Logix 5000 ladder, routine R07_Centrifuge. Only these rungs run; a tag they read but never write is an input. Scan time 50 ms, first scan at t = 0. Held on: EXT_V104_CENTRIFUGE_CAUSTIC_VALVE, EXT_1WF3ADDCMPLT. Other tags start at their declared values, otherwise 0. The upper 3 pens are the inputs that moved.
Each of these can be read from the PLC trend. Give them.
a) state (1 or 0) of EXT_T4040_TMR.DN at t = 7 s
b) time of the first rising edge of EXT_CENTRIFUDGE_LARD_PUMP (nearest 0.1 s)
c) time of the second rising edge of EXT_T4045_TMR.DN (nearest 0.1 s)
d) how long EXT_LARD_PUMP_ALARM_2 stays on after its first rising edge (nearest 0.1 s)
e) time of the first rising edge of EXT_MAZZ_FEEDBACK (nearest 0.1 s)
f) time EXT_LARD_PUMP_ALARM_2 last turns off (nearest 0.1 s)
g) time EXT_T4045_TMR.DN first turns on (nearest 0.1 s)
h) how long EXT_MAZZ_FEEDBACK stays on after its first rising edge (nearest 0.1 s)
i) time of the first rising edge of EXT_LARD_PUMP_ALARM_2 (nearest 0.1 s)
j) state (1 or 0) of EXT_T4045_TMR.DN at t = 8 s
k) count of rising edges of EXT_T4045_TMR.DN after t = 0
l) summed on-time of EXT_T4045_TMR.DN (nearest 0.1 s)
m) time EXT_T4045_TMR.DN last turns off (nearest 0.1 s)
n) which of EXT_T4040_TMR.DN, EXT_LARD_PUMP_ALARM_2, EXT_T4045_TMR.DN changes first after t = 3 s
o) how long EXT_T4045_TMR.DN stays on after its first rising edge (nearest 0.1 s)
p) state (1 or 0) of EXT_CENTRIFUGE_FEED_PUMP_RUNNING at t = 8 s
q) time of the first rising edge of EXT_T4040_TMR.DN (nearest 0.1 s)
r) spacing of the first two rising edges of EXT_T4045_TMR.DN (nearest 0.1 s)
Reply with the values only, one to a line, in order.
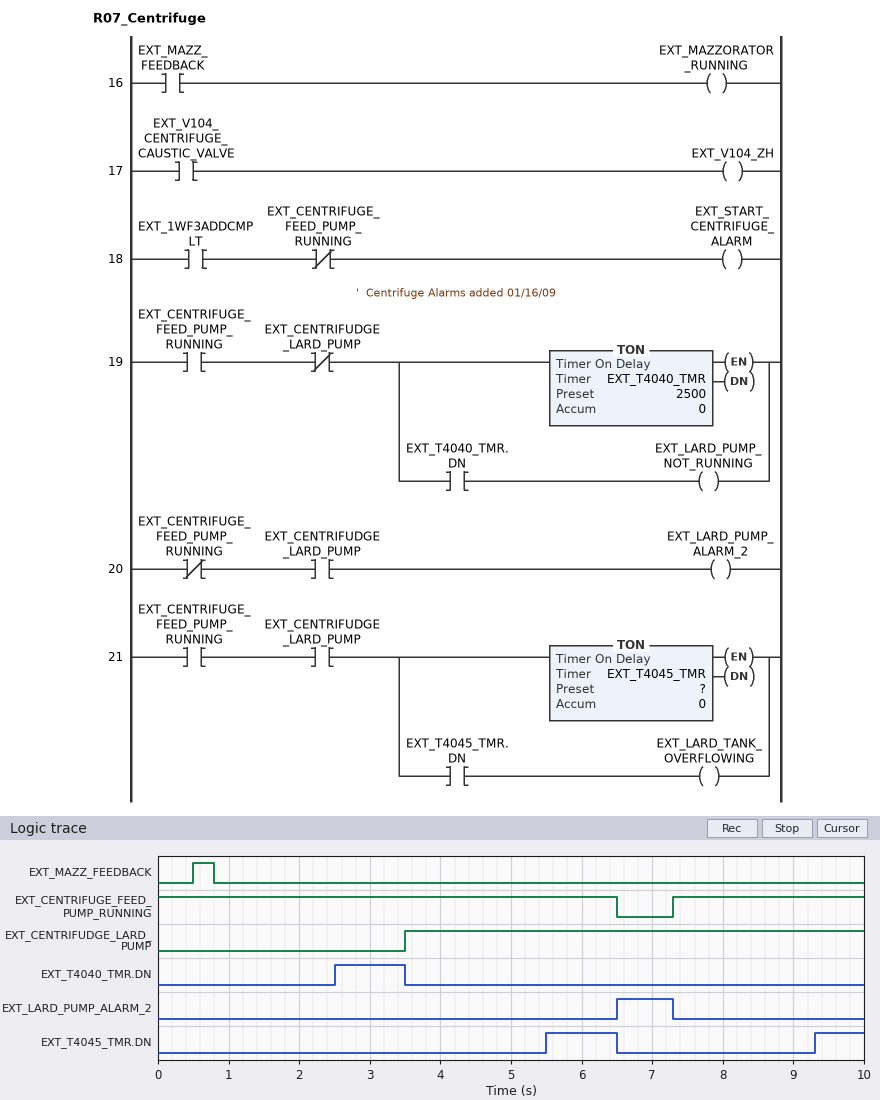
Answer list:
0
3.5 s
9.3 s
0.8 s
0.5 s
7.3 s
5.5 s
0.3 s
6.5 s
0
2
1.7 s
6.5 s
EXT_T4040_TMR.DN
1.0 s
1
2.5 s
3.8 s
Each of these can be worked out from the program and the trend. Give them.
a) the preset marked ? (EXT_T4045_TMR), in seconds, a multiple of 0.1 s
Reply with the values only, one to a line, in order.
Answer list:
2.0 s
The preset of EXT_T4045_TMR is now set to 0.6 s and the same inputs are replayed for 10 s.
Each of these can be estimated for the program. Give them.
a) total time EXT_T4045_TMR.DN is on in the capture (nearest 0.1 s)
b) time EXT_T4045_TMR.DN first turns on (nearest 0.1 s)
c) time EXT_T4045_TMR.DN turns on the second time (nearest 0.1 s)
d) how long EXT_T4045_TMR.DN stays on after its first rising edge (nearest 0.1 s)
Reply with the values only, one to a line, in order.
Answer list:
4.5 s
4.1 s
7.9 s
2.4 s
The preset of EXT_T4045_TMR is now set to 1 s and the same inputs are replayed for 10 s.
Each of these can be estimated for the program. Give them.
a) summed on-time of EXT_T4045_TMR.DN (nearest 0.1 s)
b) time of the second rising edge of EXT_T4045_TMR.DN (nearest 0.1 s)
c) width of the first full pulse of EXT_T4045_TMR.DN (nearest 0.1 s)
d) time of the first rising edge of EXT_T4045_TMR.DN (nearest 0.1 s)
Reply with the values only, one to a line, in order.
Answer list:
3.7 s
8.3 s
2.0 s
4.5 s
